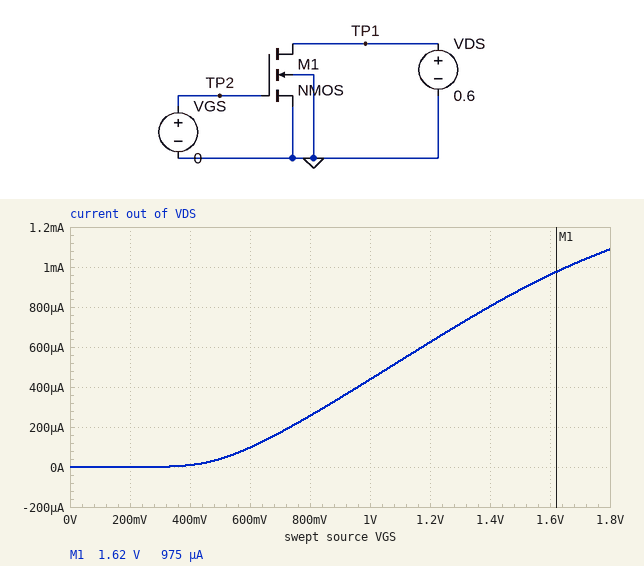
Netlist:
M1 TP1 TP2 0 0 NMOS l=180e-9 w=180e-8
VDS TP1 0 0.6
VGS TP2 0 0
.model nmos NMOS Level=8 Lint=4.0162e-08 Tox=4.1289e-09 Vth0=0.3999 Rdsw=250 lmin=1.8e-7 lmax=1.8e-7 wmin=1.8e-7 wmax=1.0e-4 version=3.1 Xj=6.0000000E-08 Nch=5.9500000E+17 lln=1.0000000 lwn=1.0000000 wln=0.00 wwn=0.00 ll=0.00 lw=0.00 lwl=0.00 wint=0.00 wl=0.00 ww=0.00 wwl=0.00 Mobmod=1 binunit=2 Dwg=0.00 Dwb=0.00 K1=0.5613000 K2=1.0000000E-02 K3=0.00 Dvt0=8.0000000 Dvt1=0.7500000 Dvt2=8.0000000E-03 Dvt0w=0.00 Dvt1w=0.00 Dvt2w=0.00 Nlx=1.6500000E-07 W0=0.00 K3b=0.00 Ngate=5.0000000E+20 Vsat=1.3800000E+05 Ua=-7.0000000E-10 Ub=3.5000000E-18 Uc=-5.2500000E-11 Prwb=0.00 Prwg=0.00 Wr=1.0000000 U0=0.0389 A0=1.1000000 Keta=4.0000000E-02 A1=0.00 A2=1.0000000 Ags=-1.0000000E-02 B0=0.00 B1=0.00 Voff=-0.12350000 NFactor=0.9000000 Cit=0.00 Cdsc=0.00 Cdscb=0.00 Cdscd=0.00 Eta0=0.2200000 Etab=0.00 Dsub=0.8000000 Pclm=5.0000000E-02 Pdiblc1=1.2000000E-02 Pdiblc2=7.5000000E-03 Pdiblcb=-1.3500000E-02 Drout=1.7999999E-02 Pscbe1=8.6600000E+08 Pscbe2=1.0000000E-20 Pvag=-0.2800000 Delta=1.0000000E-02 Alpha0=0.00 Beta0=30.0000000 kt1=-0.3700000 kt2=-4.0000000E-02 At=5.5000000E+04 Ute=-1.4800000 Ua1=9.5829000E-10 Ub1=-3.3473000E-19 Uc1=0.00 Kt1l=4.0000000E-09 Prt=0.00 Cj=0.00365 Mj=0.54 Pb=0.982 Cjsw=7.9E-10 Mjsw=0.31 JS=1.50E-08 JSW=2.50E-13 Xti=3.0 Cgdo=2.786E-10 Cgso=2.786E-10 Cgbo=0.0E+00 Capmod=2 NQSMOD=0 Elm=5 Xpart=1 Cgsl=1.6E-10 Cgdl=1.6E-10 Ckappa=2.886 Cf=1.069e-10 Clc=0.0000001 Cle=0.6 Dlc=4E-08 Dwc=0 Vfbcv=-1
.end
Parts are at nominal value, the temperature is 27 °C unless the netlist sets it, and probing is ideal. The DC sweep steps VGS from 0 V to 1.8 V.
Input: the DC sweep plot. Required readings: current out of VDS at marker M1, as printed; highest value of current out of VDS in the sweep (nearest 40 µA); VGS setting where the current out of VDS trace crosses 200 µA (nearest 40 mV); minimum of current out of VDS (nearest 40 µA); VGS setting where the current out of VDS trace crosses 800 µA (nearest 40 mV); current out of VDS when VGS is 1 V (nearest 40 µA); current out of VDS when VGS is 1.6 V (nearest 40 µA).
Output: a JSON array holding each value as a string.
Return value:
["975 µA", "1.08 mA", "720 mV", "0 A", "1.40 V", "440 µA", "960 µA"]
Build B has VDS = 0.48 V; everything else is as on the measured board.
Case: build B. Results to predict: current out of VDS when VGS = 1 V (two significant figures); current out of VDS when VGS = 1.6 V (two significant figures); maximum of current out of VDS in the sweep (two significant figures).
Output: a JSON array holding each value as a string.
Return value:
["420 µA", "870 µA", "960 µA"]
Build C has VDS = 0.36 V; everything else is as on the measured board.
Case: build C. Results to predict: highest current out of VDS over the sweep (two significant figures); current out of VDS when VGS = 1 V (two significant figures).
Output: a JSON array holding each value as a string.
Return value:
["790 µA", "390 µA"]
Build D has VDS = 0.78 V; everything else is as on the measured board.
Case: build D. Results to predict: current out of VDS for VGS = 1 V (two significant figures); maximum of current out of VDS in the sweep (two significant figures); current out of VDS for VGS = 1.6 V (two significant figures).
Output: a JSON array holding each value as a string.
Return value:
["460 µA", "1.2 mA", "1.0 mA"]
